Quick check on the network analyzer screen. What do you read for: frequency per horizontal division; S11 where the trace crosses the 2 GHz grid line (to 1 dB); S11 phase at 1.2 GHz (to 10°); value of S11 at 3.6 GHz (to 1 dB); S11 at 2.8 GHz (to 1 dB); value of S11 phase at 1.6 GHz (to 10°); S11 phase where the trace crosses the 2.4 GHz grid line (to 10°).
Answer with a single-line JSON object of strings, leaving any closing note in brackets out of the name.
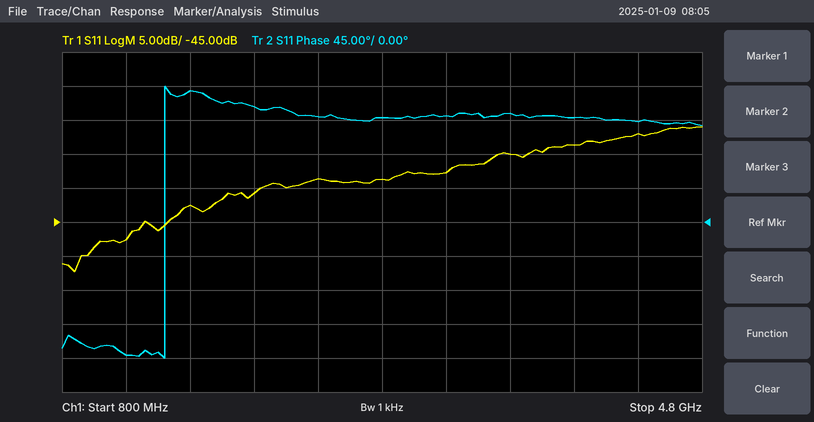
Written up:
{"frequency per horizontal division": "400 MHz", "S11 where the trace crosses the 2 GHz grid line": "-41 dB", "S11 phase at 1.2 GHz": "-180°", "value of S11 at 3.6 GHz": "-35 dB", "S11 at 2.8 GHz": "-39 dB", "value of S11 phase at 1.6 GHz": "170°", "S11 phase where the trace crosses the 2.4 GHz grid line": "140°"}
